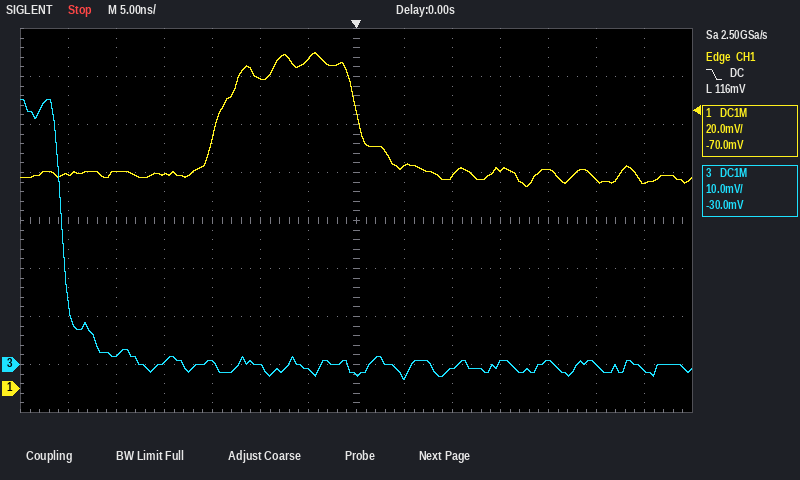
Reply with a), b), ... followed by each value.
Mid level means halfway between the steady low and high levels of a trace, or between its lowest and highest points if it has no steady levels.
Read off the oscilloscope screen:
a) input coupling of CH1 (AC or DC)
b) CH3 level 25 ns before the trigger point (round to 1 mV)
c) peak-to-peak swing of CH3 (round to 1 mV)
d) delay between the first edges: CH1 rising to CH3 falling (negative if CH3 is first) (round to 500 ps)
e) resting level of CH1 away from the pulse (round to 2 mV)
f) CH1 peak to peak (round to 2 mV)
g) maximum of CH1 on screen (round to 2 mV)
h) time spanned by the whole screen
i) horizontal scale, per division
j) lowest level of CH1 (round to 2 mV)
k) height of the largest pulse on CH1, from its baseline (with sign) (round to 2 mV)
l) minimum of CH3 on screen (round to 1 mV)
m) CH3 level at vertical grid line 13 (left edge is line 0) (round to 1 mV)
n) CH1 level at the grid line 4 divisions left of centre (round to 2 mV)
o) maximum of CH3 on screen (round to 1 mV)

a) DC
b) 2 mV
c) 58 mV
d) -16.0 ns
e) 90 mV
f) 56 mV
g) 140 mV
h) 70 ns
i) 5 ns
j) 84 mV
k) +50 mV
l) -3 mV
m) -1 mV
n) 90 mV
o) 55 mV
